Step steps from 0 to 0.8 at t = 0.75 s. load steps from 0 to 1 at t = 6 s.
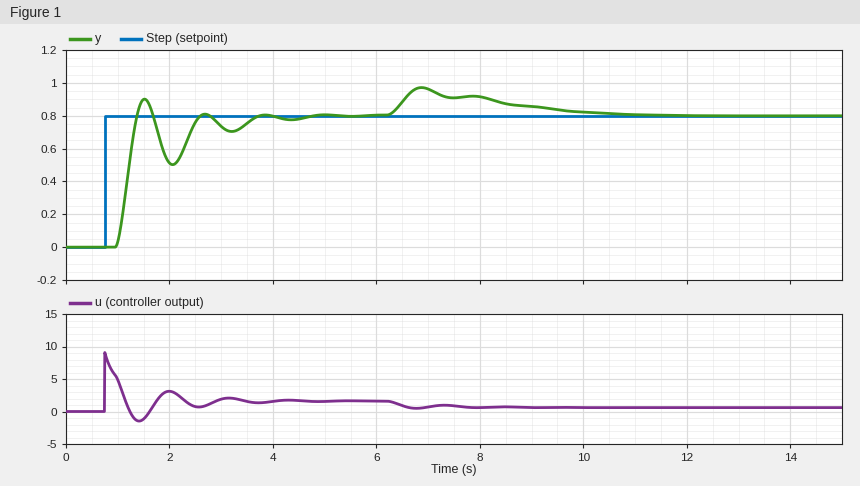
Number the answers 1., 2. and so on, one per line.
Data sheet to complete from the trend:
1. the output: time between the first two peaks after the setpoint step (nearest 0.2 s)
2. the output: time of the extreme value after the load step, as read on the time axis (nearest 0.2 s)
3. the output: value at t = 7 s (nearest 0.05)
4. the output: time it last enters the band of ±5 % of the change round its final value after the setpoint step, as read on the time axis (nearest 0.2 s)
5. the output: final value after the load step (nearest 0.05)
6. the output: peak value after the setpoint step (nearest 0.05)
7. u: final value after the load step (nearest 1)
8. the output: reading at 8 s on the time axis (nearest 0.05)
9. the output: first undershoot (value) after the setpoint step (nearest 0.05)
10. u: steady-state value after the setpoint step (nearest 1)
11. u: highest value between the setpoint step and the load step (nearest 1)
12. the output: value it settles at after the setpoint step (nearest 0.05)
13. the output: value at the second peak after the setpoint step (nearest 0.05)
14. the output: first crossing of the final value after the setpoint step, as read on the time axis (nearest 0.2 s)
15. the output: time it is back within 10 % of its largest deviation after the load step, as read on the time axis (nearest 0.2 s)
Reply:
1. 1.2 s
2. 6.8 s
3. 0.95
4. 3.6 s
5. 0.80
6. 0.90
7. 1
8. 0.90
9. 0.50
10. 2
11. 9
12. 0.80
13. 0.80
14. 1.4 s
15. 10.4 s
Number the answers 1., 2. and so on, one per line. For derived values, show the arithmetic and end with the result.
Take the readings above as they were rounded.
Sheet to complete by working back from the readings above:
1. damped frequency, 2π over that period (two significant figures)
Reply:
1. 2π / 1.2 = 5.2 rad/s
